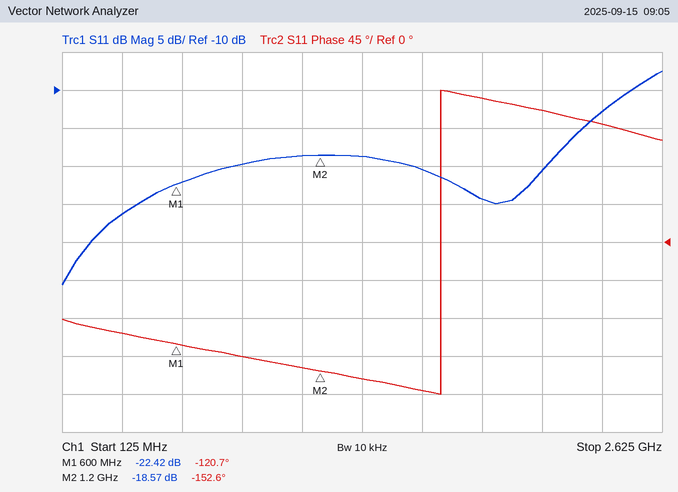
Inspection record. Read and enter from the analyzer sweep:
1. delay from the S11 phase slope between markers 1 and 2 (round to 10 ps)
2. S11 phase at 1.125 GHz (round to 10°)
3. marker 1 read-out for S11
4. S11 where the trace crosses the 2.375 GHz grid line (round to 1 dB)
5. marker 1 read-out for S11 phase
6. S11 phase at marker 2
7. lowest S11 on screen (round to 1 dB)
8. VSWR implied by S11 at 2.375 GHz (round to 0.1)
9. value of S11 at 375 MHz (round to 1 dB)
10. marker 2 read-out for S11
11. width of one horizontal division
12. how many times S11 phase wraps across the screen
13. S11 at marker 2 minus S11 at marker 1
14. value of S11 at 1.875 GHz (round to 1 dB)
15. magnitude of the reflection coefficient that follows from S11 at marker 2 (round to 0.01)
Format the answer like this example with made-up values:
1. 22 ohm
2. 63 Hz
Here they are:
1. 150 ps
2. -150°
3. -22.42 dB
4. -13 dB
5. -120.7°
6. -152.6°
7. -36 dB
8. 1.6
9. -26 dB
10. -18.57 dB
11. 250 MHz
12. 1
13. 3.85 dB
14. -24 dB
15. 0.12
